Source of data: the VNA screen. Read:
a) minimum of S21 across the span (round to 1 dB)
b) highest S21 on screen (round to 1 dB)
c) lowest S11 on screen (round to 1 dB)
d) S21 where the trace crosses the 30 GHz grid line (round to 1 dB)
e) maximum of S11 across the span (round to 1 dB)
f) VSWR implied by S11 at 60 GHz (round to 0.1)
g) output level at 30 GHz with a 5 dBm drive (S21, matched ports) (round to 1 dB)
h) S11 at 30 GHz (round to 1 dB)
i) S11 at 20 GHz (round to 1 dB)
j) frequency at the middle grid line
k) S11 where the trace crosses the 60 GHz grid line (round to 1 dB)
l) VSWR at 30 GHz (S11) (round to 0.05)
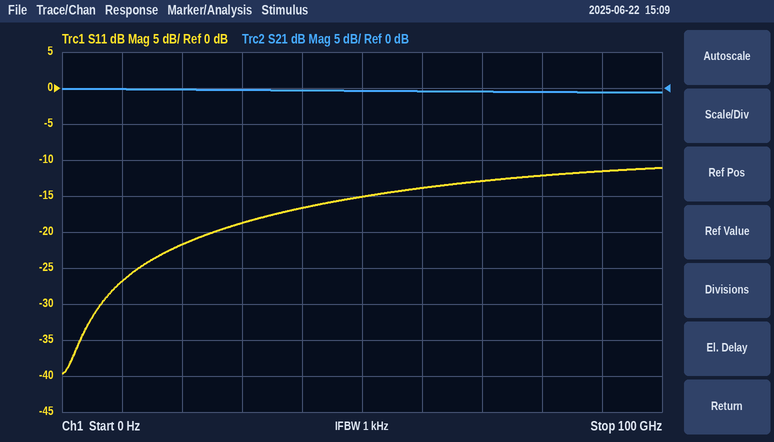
-1 dB
0 dB
-40 dB
0 dB
-11 dB
1.5
5 dBm
-19 dB
-22 dB
50 GHz
-14 dB
1.25
